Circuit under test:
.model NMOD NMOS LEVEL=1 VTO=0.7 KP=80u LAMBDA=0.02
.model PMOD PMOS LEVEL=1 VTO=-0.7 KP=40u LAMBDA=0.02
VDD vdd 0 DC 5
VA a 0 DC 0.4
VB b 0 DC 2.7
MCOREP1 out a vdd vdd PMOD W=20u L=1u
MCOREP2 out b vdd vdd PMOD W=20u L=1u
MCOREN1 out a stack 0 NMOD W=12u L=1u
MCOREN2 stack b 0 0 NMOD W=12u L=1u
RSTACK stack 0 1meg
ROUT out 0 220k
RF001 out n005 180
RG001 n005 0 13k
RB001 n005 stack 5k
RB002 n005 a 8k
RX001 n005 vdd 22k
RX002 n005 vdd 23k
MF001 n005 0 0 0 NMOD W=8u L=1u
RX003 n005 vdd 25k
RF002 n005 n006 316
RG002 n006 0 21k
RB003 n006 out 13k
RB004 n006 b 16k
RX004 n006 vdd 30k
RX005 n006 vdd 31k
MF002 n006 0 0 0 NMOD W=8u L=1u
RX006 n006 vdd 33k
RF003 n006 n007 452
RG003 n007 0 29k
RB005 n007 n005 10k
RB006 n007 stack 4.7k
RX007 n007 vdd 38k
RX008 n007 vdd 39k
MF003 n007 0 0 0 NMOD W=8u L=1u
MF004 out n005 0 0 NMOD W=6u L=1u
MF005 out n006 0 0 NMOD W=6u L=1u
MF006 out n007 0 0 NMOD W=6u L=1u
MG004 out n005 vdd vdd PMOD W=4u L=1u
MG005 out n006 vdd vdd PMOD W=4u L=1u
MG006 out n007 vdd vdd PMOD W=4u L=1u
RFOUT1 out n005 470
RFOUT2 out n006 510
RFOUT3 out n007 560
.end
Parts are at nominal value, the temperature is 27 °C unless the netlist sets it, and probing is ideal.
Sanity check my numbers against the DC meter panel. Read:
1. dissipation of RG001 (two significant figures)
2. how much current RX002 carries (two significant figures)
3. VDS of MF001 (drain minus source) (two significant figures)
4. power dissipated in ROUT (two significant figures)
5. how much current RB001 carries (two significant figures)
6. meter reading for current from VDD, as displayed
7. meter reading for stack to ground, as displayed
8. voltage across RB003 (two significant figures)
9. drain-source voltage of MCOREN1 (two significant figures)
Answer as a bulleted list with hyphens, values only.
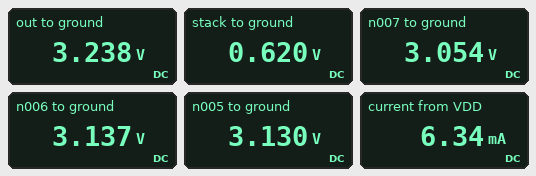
- 750 µW
- 81 µA
- 3.1 V
- 48 µW
- 500 µA
- 6.34 mA
- 0.620 V
- 100 mV
- 2.6 V
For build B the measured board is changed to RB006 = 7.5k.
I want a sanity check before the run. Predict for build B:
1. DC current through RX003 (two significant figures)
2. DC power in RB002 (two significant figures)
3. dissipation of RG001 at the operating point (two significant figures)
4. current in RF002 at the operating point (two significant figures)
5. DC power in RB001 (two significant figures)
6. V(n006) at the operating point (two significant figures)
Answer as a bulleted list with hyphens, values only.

- 74 µA
- 940 µW
- 760 µW
- 62 µA
- 1.4 mW
- 3.2 V
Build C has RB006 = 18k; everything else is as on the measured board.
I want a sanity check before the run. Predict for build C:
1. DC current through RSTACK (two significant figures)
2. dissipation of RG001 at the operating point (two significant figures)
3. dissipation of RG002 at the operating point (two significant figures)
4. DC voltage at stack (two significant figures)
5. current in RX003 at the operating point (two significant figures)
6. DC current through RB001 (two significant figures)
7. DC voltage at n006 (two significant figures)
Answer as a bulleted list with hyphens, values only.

- 400 nA
- 760 µW
- 480 µW
- 400 mV
- 74 µA
- 550 µA
- 3.2 V
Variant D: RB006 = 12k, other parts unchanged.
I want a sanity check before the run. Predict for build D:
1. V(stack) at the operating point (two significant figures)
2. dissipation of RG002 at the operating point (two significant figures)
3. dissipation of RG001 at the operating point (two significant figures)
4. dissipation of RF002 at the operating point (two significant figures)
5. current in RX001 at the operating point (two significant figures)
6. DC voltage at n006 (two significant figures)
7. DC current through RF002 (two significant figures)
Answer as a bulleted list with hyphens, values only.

- 440 mV
- 480 µW
- 760 µW
- 2.6 µW
- 84 µA
- 3.2 V
- 90 µA
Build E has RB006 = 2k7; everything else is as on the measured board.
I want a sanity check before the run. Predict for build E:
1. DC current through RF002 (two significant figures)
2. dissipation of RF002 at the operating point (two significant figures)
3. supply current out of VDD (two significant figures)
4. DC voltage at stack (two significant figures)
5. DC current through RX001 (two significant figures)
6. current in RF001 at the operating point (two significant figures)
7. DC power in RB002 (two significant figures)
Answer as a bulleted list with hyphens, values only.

- 43 µA
- 590 nW
- 6.4 mA
- 810 mV
- 86 µA
- 620 µA
- 920 µW
